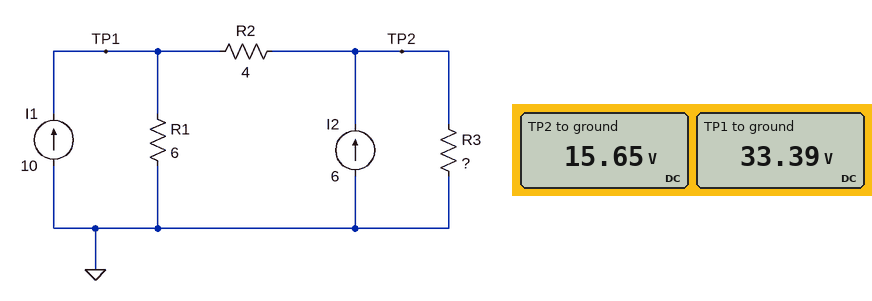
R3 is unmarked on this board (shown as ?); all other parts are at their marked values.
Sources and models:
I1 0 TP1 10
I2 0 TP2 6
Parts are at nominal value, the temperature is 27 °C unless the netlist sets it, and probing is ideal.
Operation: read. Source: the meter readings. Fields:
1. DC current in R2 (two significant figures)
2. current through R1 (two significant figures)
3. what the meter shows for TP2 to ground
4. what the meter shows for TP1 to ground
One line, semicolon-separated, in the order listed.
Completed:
4.4 A; 5.6 A; 15.65 V; 33.39 V
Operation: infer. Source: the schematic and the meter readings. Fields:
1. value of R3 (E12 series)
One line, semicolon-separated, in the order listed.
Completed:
1.5 Ω
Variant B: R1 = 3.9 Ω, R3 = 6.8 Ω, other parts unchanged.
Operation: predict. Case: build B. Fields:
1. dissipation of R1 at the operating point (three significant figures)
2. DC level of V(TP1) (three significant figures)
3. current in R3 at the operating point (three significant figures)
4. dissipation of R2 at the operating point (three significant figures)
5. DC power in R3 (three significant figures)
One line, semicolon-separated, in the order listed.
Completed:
400 W; 39.5 V; 5.88 A; 60.0 mW; 235 W
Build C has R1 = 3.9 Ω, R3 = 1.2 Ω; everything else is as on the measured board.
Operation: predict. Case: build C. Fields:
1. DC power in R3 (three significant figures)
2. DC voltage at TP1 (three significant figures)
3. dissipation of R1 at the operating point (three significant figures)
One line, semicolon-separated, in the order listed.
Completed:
108 W; 25.4 V; 165 W
